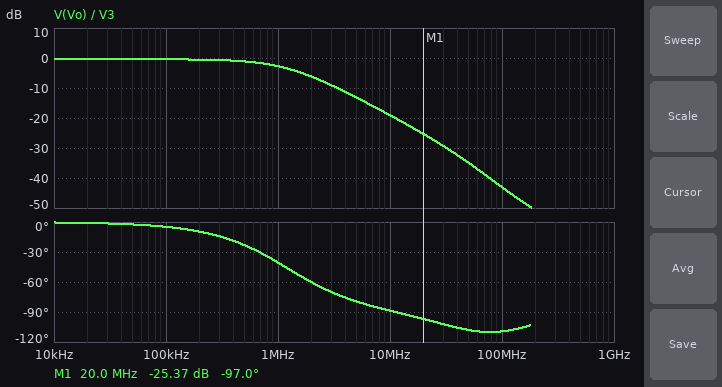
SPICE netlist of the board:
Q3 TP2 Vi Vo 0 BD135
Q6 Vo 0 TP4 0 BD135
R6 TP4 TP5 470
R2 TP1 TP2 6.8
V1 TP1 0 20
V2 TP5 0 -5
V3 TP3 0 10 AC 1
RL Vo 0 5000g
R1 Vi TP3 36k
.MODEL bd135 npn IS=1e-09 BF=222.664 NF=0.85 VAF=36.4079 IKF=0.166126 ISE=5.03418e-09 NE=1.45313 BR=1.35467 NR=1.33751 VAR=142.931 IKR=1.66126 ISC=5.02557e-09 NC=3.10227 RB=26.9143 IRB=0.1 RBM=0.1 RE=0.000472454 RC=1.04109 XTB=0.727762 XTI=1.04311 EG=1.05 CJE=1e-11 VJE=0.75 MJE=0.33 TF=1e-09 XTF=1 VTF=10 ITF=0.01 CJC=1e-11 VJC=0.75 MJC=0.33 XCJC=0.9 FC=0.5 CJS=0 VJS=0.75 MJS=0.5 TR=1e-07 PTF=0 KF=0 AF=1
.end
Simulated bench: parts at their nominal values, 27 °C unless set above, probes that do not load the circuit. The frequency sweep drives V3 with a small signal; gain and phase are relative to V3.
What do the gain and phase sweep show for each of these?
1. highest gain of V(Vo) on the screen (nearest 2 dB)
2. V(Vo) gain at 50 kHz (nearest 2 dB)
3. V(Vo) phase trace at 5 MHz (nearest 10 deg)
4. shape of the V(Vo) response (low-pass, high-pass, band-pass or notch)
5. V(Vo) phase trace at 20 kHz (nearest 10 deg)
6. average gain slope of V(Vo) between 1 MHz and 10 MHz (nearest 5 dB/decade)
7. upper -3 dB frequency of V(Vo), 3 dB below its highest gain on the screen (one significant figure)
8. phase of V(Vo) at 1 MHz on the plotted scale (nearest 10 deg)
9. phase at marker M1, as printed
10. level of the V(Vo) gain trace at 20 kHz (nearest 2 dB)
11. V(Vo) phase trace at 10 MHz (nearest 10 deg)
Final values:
0 dB
0 dB
-80 deg
low-pass
0 deg
-15 dB/decade
1 MHz
-40 deg
-97.0 deg
0 dB
-90 deg
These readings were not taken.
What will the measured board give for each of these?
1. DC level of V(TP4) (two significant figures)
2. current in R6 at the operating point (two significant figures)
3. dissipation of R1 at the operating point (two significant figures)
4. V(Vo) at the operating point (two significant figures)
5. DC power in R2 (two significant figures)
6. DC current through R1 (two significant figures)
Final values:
-350 mV
9.9 mA
270 µW
6.5 V
640 µW
86 µA
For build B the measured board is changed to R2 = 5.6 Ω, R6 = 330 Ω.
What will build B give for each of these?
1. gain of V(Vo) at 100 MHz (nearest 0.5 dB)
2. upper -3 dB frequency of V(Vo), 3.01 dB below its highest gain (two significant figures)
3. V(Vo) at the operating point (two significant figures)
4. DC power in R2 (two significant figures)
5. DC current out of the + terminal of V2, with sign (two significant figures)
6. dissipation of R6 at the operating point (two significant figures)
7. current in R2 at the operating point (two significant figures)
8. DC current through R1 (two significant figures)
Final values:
-43.5 dB
1.2 MHz
5.6 V
1.1 mW
-14 mA
65 mW
14 mA
110 µA
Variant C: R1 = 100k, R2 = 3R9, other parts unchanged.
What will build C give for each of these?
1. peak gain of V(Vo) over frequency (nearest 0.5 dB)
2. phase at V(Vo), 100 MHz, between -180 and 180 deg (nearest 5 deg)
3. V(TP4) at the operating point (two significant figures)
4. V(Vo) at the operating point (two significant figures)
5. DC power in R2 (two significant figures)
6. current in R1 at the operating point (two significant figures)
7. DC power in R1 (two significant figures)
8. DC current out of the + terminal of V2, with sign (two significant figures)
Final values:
-1.0 dB
-115 deg
-360 mV
1.6 V
370 µW
80 µA
640 µW
-9.9 mA
